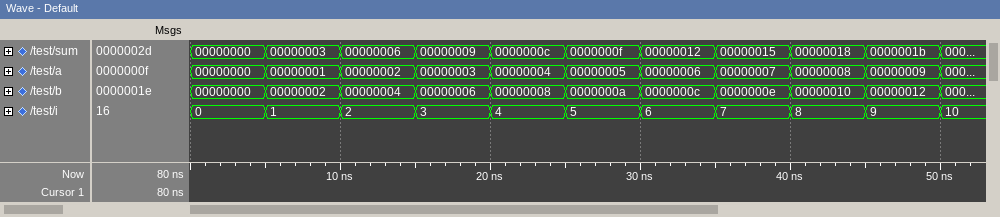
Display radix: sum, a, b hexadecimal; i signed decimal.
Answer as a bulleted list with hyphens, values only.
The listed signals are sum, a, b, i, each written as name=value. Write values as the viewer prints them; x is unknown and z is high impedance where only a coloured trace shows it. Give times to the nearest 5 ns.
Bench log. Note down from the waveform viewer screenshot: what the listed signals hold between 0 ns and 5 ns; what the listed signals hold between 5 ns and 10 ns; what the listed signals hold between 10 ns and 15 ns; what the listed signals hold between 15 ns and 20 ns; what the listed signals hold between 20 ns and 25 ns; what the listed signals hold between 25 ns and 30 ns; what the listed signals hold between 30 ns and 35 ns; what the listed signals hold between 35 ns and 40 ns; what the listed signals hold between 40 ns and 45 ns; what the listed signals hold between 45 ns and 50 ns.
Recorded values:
- sum=00000000, a=00000000, b=00000000, i=0
- sum=00000003, a=00000001, b=00000002, i=1
- sum=00000006, a=00000002, b=00000004, i=2
- sum=00000009, a=00000003, b=00000006, i=3
- sum=0000000c, a=00000004, b=00000008, i=4
- sum=0000000f, a=00000005, b=0000000a, i=5
- sum=00000012, a=00000006, b=0000000c, i=6
- sum=00000015, a=00000007, b=0000000e, i=7
- sum=00000018, a=00000008, b=00000010, i=8
- sum=0000001b, a=00000009, b=00000012, i=9
